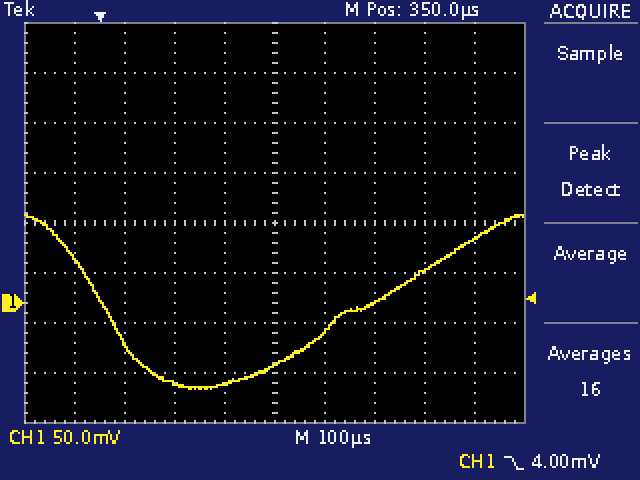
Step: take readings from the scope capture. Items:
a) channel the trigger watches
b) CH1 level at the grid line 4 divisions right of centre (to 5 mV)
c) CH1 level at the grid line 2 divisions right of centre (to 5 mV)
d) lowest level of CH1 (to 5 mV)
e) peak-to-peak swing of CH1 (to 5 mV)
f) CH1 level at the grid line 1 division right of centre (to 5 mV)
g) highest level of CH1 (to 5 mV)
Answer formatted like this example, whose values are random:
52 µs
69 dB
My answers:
CH1
65 mV
0 mV
-85 mV
175 mV
-30 mV
90 mV
